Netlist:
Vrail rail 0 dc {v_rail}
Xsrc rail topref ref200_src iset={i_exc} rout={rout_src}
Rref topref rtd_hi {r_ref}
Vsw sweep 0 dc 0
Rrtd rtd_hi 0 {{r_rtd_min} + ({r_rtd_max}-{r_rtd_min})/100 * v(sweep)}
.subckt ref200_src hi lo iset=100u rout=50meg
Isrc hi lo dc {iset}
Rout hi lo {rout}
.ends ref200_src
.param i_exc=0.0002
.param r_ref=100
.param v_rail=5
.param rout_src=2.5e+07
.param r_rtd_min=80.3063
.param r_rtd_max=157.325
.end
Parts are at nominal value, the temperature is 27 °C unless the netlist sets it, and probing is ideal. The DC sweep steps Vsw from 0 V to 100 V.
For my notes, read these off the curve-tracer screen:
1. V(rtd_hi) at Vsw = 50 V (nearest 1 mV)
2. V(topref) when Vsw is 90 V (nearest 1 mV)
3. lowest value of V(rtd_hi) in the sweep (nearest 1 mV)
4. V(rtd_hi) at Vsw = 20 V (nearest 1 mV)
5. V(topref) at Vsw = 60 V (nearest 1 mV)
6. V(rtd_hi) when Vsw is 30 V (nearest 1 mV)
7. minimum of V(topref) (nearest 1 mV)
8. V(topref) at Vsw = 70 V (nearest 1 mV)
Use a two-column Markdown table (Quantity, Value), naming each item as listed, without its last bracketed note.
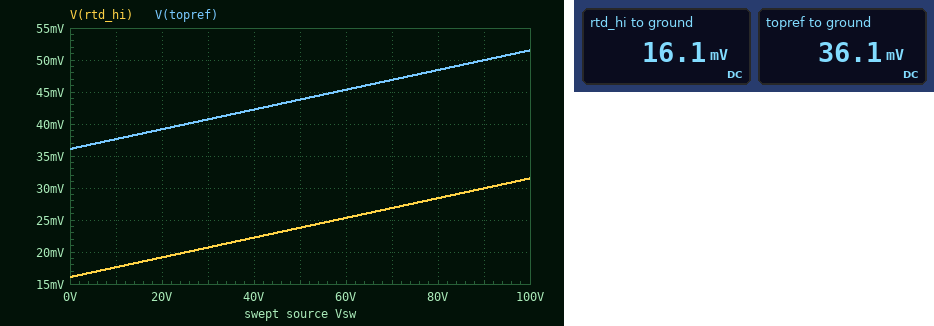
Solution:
| Quantity | Value |
|---|---|
| V(rtd_hi) at Vsw = 50 V | 24 mV |
| V(topref) when Vsw is 90 V | 50 mV |
| lowest value of V(rtd_hi) in the sweep | 16 mV |
| V(rtd_hi) at Vsw = 20 V | 19 mV |
| V(topref) at Vsw = 60 V | 45 mV |
| V(rtd_hi) when Vsw is 30 V | 21 mV |
| minimum of V(topref) | 36 mV |
| V(topref) at Vsw = 70 V | 47 mV |
